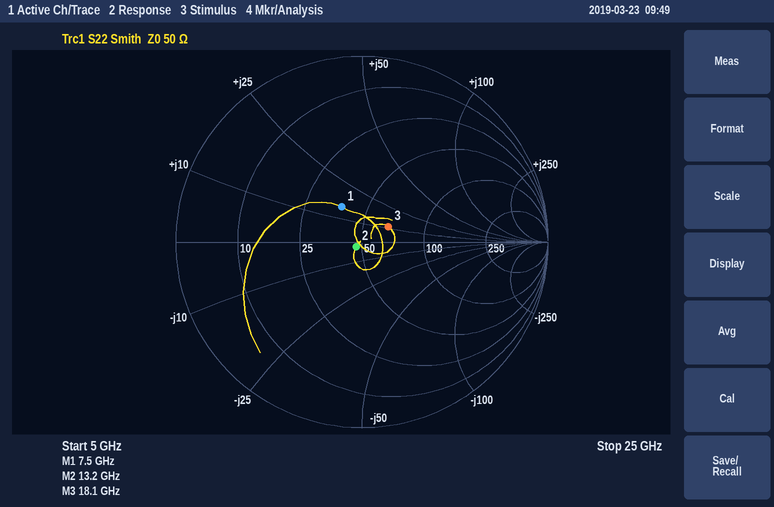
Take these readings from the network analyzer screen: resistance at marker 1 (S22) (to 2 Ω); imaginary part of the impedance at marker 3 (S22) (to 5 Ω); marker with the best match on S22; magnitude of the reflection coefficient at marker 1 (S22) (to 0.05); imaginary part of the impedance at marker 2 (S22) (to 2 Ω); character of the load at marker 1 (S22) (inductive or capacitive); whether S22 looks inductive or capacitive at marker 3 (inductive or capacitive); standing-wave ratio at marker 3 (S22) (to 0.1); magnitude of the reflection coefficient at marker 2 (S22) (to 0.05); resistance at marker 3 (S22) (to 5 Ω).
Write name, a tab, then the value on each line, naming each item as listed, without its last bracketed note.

resistance at marker 1 (S22)	38 Ω
imaginary part of the impedance at marker 3 (S22)	+10 Ω
marker with the best match on S22	marker 2
magnitude of the reflection coefficient at marker 1 (S22)	0.20
imaginary part of the impedance at marker 2 (S22)	-2 Ω
character of the load at marker 1 (S22)	inductive
whether S22 looks inductive or capacitive at marker 3	inductive
standing-wave ratio at marker 3 (S22)	1.4
magnitude of the reflection coefficient at marker 2 (S22)	0.05
resistance at marker 3 (S22)	65 Ω
